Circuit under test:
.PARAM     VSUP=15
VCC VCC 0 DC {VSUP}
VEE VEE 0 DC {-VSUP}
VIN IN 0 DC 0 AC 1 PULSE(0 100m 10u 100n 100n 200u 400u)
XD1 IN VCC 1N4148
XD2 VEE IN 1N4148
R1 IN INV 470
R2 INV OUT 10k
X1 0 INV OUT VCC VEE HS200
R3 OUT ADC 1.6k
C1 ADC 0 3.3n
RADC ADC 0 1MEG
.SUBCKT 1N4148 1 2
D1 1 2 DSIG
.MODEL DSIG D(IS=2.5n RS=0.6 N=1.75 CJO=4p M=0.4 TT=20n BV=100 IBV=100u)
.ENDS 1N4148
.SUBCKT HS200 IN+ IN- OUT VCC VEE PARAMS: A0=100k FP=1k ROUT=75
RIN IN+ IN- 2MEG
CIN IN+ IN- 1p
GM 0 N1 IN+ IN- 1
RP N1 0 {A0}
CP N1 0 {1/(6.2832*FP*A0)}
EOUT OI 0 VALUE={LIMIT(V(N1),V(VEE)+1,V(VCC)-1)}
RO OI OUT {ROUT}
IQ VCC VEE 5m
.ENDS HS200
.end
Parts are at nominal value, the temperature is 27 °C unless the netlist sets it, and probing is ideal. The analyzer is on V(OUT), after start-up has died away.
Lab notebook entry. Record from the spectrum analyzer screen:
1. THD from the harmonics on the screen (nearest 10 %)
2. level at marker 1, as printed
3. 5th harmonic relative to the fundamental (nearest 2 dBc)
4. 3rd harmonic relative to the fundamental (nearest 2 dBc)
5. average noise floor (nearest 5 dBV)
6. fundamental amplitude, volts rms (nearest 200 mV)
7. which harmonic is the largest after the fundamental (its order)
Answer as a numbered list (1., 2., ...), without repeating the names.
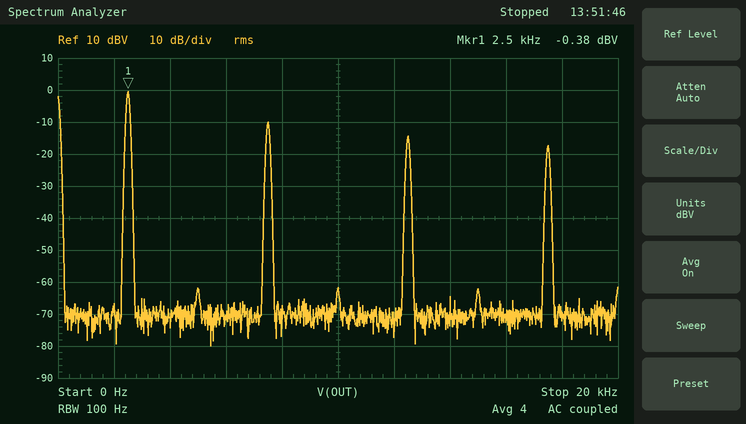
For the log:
1. 40 %
2. -0.38 dBV
3. -14 dBc
4. -10 dBc
5. -70 dBV
6. 1.0 V
7. 3
